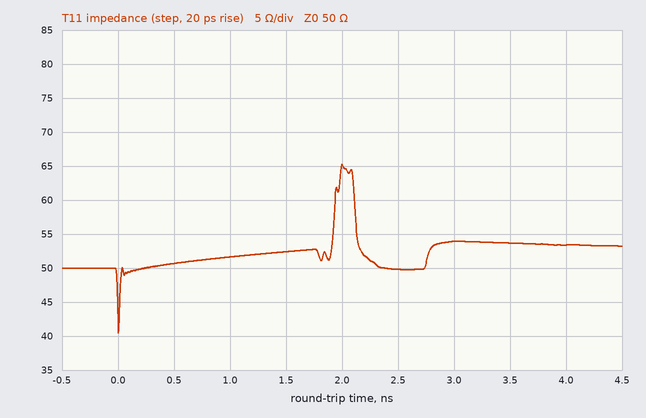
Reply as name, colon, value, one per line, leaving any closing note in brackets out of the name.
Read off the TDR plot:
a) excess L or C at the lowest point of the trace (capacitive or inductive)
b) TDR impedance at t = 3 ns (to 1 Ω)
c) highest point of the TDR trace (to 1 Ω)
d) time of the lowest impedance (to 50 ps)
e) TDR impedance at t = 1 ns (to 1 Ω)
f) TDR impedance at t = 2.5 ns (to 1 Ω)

excess L or C at the lowest point of the trace: capacitive
TDR impedance at t = 3 ns: 54 Ω
highest point of the TDR trace: 65 Ω
time of the lowest impedance: 0 ps
TDR impedance at t = 1 ns: 52 Ω
TDR impedance at t = 2.5 ns: 50 Ω
